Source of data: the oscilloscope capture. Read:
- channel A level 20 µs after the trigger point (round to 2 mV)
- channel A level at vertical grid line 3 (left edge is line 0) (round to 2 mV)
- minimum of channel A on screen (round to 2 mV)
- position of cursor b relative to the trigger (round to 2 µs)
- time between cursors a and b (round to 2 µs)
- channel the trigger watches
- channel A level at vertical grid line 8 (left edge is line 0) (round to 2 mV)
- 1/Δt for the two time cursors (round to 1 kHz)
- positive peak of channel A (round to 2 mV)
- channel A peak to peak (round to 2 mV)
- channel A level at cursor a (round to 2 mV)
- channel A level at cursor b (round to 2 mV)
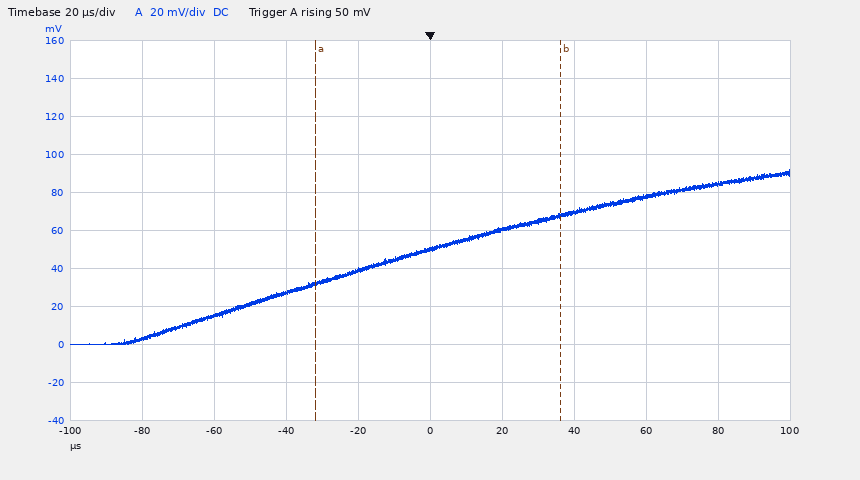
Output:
60 mV
28 mV
0 mV
+36 µs
68 µs
channel A
78 mV
15 kHz
92 mV
92 mV
32 mV
68 mV
